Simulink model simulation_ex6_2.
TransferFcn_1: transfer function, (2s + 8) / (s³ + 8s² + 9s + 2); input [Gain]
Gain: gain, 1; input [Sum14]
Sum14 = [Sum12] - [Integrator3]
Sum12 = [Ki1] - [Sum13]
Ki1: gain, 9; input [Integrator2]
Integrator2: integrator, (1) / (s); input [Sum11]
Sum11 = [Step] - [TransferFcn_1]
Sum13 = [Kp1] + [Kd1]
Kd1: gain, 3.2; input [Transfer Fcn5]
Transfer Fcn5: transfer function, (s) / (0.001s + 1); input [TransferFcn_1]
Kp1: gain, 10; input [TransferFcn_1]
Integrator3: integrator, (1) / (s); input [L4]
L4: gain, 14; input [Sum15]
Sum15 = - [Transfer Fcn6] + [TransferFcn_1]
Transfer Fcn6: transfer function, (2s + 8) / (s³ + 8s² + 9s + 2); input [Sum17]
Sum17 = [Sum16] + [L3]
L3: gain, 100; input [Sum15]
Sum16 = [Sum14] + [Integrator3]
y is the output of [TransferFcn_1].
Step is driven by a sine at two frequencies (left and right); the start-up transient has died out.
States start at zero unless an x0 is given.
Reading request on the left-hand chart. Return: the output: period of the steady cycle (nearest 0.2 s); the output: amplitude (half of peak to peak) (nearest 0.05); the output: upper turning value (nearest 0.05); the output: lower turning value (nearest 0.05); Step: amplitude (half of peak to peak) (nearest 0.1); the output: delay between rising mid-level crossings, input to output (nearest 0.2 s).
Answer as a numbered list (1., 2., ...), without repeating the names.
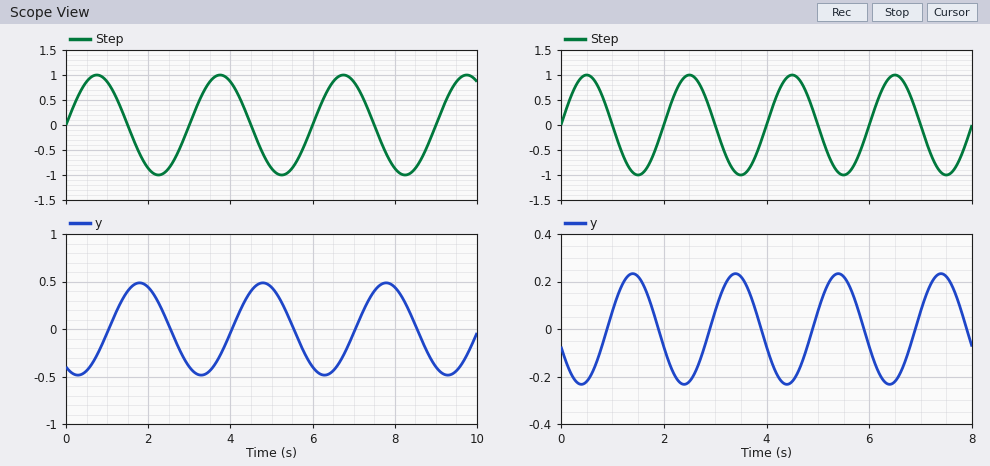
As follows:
1. 3.0 s
2. 0.50
3. 0.50
4. -0.50
5. 1.0
6. 1.0 s
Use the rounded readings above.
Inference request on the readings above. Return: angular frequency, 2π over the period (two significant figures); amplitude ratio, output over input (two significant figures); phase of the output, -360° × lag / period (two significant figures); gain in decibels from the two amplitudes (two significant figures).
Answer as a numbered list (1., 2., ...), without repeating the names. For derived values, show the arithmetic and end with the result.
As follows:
1. 2π / 3 = 2.1 rad/s
2. 0.5 / 1 = 0.50
3. -360 × 1 / 3 = -120°
4. 20 log10(0.5 / 1) = -6.0 dB
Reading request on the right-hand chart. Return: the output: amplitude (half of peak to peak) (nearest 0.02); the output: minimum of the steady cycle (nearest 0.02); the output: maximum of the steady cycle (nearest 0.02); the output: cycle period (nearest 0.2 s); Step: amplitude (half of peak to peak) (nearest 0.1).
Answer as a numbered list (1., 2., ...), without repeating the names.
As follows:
1. 0.24
2. -0.24
3. 0.24
4. 2.0 s
5. 1.0
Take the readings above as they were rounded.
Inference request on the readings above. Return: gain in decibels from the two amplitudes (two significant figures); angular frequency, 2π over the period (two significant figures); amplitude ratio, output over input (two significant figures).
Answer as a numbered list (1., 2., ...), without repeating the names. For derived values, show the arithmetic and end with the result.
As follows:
1. 20 log10(0.24 / 1) = -12 dB
2. 2π / 2 = 3.1 rad/s
3. 0.24 / 1 = 0.24
